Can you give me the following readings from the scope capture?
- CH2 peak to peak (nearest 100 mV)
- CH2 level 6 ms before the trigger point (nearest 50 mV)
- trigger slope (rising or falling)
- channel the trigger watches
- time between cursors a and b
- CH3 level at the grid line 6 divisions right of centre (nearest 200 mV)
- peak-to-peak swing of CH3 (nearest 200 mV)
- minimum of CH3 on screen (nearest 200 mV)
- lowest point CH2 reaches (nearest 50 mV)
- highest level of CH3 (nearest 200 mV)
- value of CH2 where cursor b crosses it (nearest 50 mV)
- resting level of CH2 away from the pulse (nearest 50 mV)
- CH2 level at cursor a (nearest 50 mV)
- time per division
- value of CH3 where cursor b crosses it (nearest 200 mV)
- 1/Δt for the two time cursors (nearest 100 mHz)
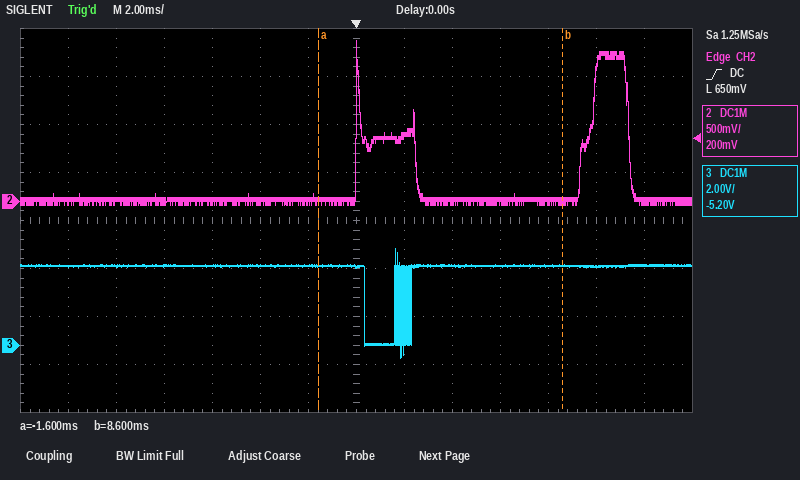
1.70 V
0 mV
rising
CH2
10.2 ms
3.4 V
4.6 V
-600 mV
-50 mV
4.0 V
0 mV
0 mV
0 mV
2 ms
3.4 V
98.0 Hz
